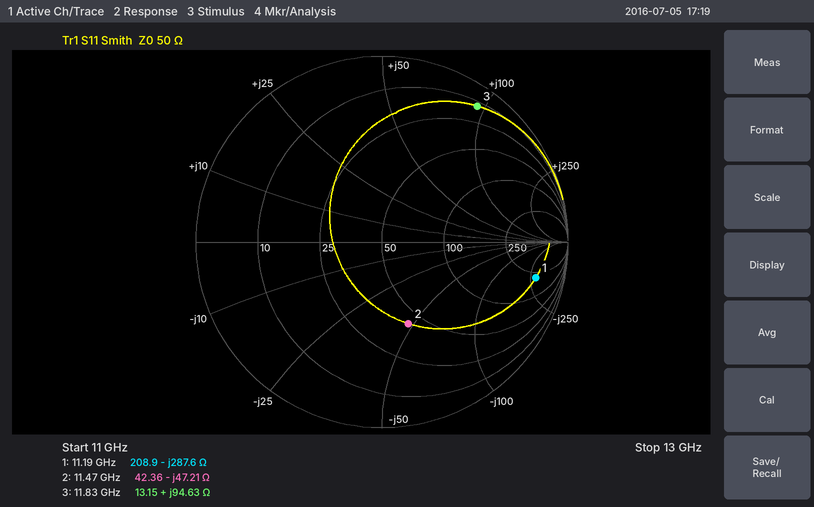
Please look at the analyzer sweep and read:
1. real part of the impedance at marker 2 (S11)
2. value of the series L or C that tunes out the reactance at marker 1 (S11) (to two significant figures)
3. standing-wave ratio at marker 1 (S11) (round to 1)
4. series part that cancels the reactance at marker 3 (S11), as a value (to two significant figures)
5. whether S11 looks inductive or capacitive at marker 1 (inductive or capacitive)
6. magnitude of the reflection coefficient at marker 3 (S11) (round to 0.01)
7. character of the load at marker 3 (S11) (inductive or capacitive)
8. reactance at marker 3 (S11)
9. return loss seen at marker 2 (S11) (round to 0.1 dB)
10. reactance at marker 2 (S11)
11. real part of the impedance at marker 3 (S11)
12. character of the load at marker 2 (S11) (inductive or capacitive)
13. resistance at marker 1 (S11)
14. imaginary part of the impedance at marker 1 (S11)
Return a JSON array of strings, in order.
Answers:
["42.36 Ω", "4.1 nH", "12", "140 fF", "capacitive", "0.89", "inductive", "+94.63 Ω", "6.7 dB", "-47.21 Ω", "13.15 Ω", "capacitive", "208.9 Ω", "-287.6 Ω"]
